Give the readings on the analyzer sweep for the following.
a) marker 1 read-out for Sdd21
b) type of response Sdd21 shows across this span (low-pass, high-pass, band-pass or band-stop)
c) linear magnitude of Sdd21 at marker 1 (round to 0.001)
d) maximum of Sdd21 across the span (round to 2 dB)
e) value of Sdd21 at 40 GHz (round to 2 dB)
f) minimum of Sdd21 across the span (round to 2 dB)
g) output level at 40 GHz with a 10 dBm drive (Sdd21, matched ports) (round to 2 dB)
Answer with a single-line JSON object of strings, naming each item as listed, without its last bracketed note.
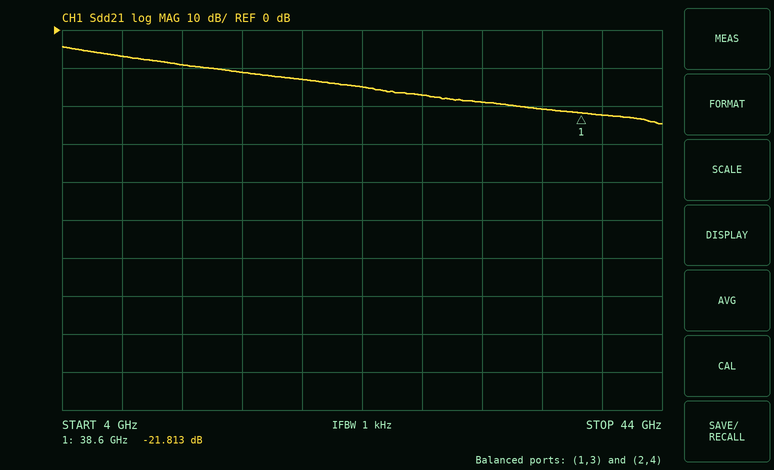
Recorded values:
{"marker 1 read-out for Sdd21": "-21.813 dB", "type of response Sdd21 shows across this span": "low-pass", "linear magnitude of Sdd21 at marker 1": "0.081", "maximum of Sdd21 across the span": "-4 dB", "value of Sdd21 at 40 GHz": "-22 dB", "minimum of Sdd21 across the span": "-24 dB", "output level at 40 GHz with a 10 dBm drive (Sdd21, matched ports)": "-12 dBm"}
